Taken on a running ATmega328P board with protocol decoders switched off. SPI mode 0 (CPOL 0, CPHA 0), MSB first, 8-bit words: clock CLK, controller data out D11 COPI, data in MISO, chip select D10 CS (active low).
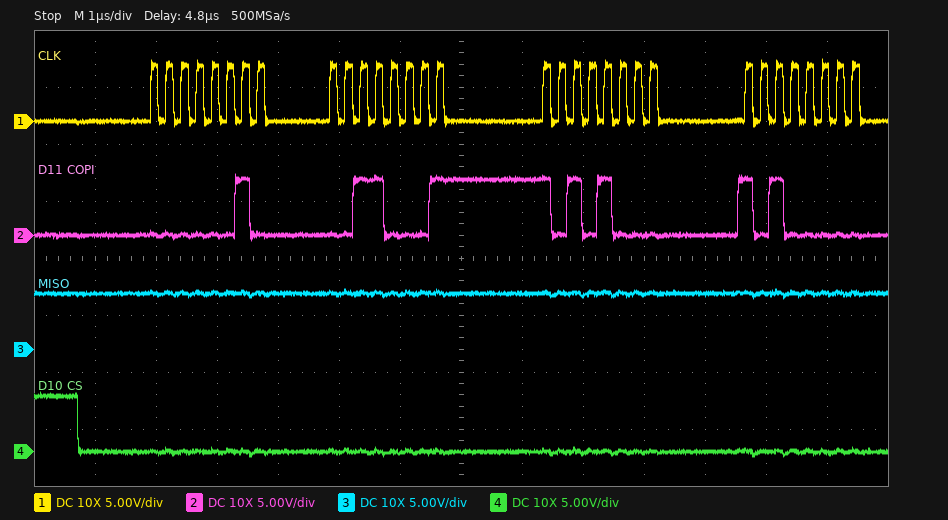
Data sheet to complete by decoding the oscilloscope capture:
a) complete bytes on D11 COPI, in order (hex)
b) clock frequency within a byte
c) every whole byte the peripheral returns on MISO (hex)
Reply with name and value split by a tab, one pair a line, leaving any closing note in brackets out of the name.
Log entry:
complete bytes on D11 COPI, in order	02 31 A8 A0
clock frequency within a byte	4 MHz
every whole byte the peripheral returns on MISO	FF FF FF FF
